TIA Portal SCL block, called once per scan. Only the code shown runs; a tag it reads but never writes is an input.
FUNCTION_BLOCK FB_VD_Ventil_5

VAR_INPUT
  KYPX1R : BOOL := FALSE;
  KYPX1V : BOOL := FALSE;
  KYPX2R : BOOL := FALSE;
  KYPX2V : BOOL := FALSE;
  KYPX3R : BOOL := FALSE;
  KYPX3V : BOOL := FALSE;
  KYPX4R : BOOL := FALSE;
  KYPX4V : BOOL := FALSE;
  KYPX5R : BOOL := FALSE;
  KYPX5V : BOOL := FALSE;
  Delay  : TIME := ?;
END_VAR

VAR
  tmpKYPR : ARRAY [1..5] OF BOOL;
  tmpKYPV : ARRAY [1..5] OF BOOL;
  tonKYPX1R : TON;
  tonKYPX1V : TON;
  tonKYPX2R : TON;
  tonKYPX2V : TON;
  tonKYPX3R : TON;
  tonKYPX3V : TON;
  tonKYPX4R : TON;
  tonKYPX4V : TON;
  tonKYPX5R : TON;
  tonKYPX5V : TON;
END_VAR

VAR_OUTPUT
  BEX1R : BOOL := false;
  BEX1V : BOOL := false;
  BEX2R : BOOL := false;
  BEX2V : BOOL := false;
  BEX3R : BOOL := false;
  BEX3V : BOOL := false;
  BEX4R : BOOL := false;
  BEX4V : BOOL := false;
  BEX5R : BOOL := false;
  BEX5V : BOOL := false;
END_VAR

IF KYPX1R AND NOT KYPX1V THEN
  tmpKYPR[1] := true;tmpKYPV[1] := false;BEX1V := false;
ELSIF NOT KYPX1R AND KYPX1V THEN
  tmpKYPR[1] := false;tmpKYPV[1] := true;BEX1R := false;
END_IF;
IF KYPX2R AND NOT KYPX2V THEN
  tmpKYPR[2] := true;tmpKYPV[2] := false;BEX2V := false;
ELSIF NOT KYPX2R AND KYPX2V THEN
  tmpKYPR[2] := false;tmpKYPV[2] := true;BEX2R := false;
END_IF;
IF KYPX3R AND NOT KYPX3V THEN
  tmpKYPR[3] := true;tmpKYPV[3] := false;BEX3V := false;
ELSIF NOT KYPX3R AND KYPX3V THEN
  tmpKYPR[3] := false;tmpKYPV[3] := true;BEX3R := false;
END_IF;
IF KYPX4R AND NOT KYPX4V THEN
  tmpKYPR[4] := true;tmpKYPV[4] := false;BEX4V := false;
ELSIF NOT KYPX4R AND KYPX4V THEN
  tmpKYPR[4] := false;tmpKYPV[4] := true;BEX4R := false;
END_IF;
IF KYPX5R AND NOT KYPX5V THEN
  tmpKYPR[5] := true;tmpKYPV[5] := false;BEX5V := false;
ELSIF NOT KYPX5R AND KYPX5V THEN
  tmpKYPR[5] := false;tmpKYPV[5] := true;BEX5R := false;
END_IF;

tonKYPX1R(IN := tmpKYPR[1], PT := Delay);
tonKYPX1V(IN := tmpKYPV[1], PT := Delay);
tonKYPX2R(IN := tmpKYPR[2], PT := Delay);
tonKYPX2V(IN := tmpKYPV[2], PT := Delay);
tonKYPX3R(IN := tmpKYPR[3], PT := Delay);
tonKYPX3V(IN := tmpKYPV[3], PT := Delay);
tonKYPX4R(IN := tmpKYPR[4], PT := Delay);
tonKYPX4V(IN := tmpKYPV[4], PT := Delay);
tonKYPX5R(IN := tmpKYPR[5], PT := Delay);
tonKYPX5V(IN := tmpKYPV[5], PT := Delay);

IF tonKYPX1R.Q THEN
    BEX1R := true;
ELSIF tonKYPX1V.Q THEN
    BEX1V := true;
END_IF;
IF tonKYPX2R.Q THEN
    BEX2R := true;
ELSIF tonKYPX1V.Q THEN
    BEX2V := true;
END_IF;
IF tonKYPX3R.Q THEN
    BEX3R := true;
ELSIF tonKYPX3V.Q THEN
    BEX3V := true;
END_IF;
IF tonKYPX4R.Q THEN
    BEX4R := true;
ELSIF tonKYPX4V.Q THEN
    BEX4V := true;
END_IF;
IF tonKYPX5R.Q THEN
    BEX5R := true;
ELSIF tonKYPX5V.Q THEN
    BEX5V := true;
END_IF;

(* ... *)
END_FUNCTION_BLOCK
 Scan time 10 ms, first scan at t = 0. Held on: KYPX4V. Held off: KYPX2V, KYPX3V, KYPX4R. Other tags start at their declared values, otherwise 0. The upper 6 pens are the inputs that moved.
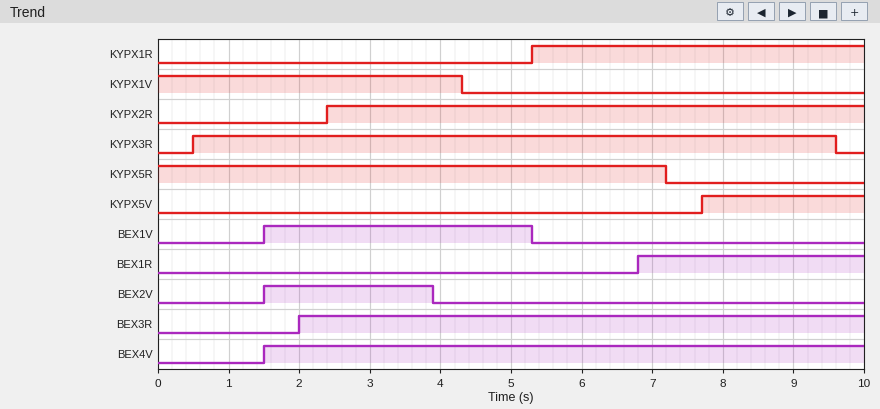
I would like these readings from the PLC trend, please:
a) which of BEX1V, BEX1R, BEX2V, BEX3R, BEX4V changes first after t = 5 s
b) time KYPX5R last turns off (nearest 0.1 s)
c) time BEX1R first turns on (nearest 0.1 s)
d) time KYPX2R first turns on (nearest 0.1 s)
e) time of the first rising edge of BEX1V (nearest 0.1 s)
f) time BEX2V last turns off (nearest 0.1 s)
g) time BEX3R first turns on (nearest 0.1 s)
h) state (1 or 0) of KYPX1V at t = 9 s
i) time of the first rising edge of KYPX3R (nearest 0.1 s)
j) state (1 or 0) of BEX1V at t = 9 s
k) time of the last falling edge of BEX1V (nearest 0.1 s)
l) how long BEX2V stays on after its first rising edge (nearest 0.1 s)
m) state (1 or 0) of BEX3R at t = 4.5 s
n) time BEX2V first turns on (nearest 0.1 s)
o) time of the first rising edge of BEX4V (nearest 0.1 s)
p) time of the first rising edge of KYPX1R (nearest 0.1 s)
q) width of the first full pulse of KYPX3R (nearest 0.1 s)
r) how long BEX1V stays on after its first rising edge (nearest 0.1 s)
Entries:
BEX1V
7.2 s
6.8 s
2.4 s
1.5 s
3.9 s
2.0 s
0
0.5 s
0
5.3 s
2.4 s
1
1.5 s
1.5 s
5.3 s
9.1 s
3.8 s
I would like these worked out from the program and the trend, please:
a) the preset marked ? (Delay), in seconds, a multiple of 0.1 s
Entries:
1.5 s
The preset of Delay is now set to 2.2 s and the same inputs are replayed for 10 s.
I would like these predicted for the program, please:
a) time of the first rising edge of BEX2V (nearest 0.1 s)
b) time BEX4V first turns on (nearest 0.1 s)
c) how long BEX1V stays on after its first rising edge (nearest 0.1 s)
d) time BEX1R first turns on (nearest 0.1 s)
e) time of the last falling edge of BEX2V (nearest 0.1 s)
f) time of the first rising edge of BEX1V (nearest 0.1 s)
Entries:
2.2 s
2.2 s
3.1 s
7.5 s
4.6 s
2.2 s
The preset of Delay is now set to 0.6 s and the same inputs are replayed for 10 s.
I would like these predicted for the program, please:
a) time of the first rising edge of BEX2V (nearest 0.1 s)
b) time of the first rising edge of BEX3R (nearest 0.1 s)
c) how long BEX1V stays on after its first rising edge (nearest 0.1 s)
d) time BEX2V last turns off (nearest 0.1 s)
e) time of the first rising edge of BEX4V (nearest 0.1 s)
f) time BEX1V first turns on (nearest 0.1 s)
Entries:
0.6 s
1.1 s
4.7 s
3.0 s
0.6 s
0.6 s
